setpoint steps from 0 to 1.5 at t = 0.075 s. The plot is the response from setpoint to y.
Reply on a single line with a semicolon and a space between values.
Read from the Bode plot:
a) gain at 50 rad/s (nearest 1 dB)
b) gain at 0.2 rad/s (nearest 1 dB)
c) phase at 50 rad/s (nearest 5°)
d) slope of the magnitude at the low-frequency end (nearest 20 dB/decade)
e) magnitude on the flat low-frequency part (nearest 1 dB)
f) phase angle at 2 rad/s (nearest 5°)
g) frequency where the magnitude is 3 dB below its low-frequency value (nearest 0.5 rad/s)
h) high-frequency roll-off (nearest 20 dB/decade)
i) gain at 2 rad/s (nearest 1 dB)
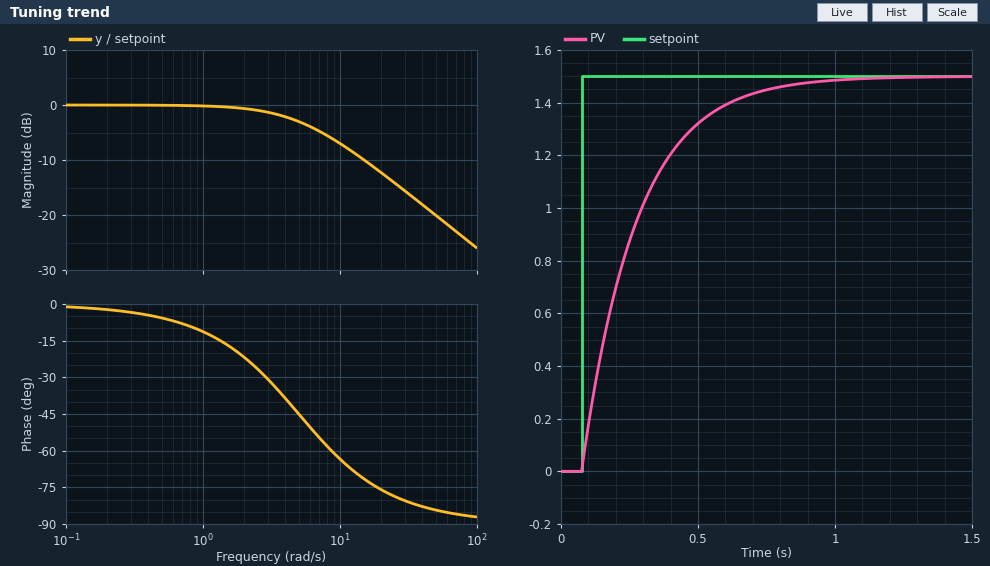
-20 dB; 0 dB; -85°; 0 dB/decade; 0 dB; -20°; 5.0 rad/s; -20 dB/decade; -1 dB
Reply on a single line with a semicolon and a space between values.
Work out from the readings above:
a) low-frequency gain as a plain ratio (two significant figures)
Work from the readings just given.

1.0
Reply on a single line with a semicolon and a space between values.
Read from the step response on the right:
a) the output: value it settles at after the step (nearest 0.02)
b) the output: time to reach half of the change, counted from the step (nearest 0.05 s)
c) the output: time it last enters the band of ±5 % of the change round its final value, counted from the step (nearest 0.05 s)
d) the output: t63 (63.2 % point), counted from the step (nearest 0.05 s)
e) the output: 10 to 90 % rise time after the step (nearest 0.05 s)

1.50; 0.15 s; 0.60 s; 0.20 s; 0.45 s
